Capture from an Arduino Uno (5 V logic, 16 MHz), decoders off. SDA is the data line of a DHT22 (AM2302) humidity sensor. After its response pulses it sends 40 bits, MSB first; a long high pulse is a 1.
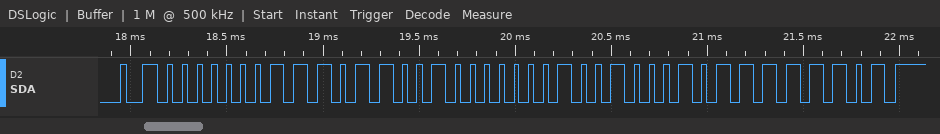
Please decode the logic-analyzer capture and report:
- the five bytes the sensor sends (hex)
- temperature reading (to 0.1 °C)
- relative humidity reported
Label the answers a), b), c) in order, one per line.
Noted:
a) 01 D9 01 22 FD
b) 29.0 °C
c) 47.3 %
